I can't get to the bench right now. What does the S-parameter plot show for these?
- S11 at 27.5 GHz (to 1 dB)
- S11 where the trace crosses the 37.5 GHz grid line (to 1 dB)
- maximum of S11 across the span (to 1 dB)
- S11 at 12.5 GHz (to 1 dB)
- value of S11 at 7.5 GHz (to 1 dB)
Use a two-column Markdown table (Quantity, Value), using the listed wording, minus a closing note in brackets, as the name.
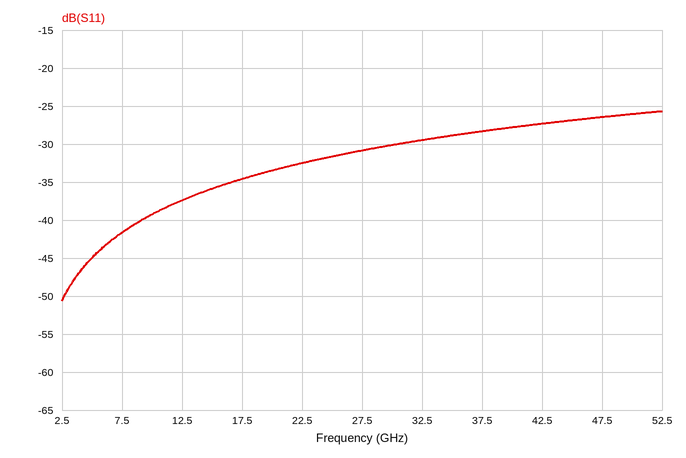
| Quantity | Value |
|---|---|
| S11 at 27.5 GHz | -31 dB |
| S11 where the trace crosses the 37.5 GHz grid line | -28 dB |
| maximum of S11 across the span | -26 dB |
| S11 at 12.5 GHz | -37 dB |
| value of S11 at 7.5 GHz | -42 dB |
